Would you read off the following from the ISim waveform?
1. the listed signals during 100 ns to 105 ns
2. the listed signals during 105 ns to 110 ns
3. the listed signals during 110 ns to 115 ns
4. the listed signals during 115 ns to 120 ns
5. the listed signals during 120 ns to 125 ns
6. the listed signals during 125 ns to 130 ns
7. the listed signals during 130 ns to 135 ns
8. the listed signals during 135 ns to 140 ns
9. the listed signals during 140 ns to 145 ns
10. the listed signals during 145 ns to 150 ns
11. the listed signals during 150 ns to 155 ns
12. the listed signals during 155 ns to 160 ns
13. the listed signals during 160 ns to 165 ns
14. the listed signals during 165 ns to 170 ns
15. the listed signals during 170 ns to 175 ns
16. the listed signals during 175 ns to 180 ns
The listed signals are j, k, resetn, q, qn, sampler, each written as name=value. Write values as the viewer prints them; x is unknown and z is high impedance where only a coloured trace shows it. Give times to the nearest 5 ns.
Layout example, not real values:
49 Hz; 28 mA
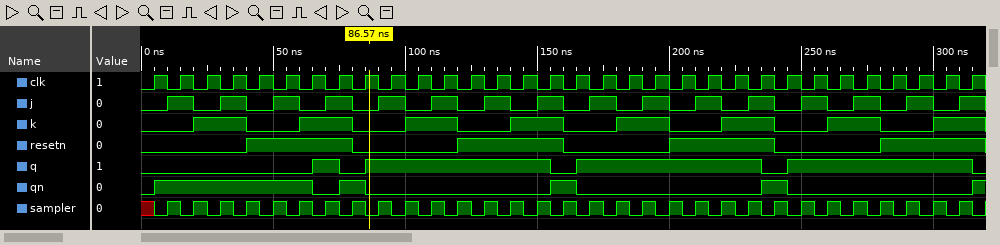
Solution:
j=0, k=1, resetn=0, q=1, qn=0, sampler=1; j=0, k=1, resetn=0, q=1, qn=0, sampler=0; j=1, k=1, resetn=0, q=1, qn=0, sampler=1; j=1, k=1, resetn=0, q=1, qn=0, sampler=0; j=0, k=0, resetn=1, q=1, qn=0, sampler=1; j=0, k=0, resetn=1, q=1, qn=0, sampler=0; j=1, k=0, resetn=1, q=1, qn=0, sampler=1; j=1, k=0, resetn=1, q=1, qn=0, sampler=0; j=0, k=1, resetn=1, q=1, qn=0, sampler=1; j=0, k=1, resetn=1, q=1, qn=0, sampler=0; j=1, k=1, resetn=1, q=1, qn=0, sampler=1; j=1, k=1, resetn=1, q=0, qn=1, sampler=0; j=0, k=0, resetn=0, q=0, qn=1, sampler=1; j=0, k=0, resetn=0, q=1, qn=0, sampler=0; j=1, k=0, resetn=0, q=1, qn=0, sampler=1; j=1, k=0, resetn=0, q=1, qn=0, sampler=0
